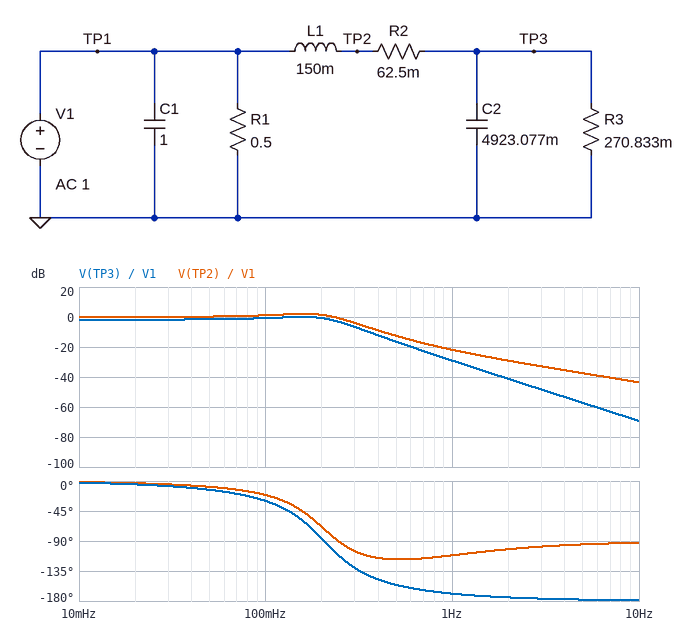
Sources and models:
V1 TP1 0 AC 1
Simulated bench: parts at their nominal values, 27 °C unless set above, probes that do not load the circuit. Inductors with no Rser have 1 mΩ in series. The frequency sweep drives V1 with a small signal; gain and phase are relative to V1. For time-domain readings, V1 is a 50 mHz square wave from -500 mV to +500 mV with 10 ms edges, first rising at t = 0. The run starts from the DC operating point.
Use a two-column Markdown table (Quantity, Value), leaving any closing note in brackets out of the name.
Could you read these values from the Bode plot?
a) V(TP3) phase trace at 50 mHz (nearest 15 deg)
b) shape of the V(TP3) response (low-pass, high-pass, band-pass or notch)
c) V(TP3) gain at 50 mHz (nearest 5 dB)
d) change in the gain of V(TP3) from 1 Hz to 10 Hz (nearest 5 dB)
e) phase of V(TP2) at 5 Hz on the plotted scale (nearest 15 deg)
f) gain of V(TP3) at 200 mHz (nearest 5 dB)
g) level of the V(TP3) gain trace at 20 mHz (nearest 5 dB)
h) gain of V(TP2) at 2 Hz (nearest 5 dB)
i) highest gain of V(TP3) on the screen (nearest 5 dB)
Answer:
| Quantity | Value |
|---|---|
| V(TP3) phase trace at 50 mHz | -15 deg |
| shape of the V(TP3) response | low-pass |
| V(TP3) gain at 50 mHz | 0 dB |
| change in the gain of V(TP3) from 1 Hz to 10 Hz | -40 dB |
| phase of V(TP2) at 5 Hz on the plotted scale | -90 deg |
| gain of V(TP3) at 200 mHz | 0 dB |
| level of the V(TP3) gain trace at 20 mHz | 0 dB |
| gain of V(TP2) at 2 Hz | -30 dB |
| highest gain of V(TP3) on the screen | 0 dB |
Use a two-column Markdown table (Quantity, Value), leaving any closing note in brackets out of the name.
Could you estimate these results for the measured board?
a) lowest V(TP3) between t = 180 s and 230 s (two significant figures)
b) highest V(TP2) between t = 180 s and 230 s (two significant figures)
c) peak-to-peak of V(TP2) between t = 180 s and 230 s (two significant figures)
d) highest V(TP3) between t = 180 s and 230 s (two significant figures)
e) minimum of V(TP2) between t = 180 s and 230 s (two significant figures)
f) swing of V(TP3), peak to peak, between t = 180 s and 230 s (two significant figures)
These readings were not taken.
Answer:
| Quantity | Value |
|---|---|
| lowest V(TP3) between t = 180 s and 230 s | -570 mV |
| highest V(TP2) between t = 180 s and 230 s | 710 mV |
| peak-to-peak of V(TP2) between t = 180 s and 230 s | 1.4 V |
| highest V(TP3) between t = 180 s and 230 s | 570 mV |
| minimum of V(TP2) between t = 180 s and 230 s | -710 mV |
| swing of V(TP3), peak to peak, between t = 180 s and 230 s | 1.1 V |
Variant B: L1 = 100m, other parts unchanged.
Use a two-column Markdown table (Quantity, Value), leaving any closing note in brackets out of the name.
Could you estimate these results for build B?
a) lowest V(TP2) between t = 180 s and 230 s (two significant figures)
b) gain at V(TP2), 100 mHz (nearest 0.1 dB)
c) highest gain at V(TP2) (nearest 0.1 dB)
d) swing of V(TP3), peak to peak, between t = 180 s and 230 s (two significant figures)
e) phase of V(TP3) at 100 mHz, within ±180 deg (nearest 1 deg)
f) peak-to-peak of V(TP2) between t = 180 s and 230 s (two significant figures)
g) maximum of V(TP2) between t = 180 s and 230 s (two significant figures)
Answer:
| Quantity | Value |
|---|---|
| lowest V(TP2) between t = 180 s and 230 s | -740 mV |
| gain at V(TP2), 100 mHz | 0.9 dB |
| highest gain at V(TP2) | 2.5 dB |
| swing of V(TP3), peak to peak, between t = 180 s and 230 s | 1.2 V |
| phase of V(TP3) at 100 mHz, within ±180 deg | -22 deg |
| peak-to-peak of V(TP2) between t = 180 s and 230 s | 1.5 V |
| maximum of V(TP2) between t = 180 s and 230 s | 740 mV |
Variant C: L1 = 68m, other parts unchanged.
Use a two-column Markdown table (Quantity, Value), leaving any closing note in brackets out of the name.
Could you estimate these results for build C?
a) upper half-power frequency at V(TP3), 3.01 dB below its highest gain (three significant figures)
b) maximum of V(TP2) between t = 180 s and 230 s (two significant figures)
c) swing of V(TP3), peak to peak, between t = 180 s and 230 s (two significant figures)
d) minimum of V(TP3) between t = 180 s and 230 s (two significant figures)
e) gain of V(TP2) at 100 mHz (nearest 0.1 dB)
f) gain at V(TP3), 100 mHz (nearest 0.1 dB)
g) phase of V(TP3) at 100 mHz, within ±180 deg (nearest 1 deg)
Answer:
| Quantity | Value |
|---|---|
| upper half-power frequency at V(TP3), 3.01 dB below its highest gain | 362 mHz |
| maximum of V(TP2) between t = 180 s and 230 s | 750 mV |
| swing of V(TP3), peak to peak, between t = 180 s and 230 s | 1.2 V |
| minimum of V(TP3) between t = 180 s and 230 s | -580 mV |
| gain of V(TP2) at 100 mHz | 0.6 dB |
| gain at V(TP3), 100 mHz | -1.3 dB |
| phase of V(TP3) at 100 mHz, within ±180 deg | -18 deg |
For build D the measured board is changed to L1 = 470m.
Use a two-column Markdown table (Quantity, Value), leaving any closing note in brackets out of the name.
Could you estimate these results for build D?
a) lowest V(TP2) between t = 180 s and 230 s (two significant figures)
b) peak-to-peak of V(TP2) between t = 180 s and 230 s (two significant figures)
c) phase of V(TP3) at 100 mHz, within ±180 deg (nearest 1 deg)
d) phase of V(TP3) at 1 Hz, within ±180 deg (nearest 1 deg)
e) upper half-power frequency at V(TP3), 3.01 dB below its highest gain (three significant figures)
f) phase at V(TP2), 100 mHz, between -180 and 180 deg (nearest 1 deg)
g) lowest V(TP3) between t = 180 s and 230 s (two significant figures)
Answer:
| Quantity | Value |
|---|---|
| lowest V(TP2) between t = 180 s and 230 s | -590 mV |
| peak-to-peak of V(TP2) between t = 180 s and 230 s | 1.2 V |
| phase of V(TP3) at 100 mHz, within ±180 deg | -76 deg |
| phase of V(TP3) at 1 Hz, within ±180 deg | -172 deg |
| upper half-power frequency at V(TP3), 3.01 dB below its highest gain | 129 mHz |
| phase at V(TP2), 100 mHz, between -180 and 180 deg | -67 deg |
| lowest V(TP3) between t = 180 s and 230 s | -480 mV |
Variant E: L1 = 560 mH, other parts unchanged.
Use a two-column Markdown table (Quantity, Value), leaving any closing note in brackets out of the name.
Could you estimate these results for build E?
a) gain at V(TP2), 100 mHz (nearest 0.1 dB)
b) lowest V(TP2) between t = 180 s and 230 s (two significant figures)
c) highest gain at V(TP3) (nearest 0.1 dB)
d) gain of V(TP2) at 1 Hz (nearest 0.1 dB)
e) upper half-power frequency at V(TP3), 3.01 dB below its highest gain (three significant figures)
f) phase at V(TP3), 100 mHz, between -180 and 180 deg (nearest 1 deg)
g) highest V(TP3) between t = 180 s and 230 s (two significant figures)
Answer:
| Quantity | Value |
|---|---|
| gain at V(TP2), 100 mHz | -1.6 dB |
| lowest V(TP2) between t = 180 s and 230 s | -570 mV |
| highest gain at V(TP3) | -1.7 dB |
| gain of V(TP2) at 1 Hz | -33.5 dB |
| upper half-power frequency at V(TP3), 3.01 dB below its highest gain | 114 mHz |
| phase at V(TP3), 100 mHz, between -180 and 180 deg | -84 deg |
| highest V(TP3) between t = 180 s and 230 s | 460 mV |
